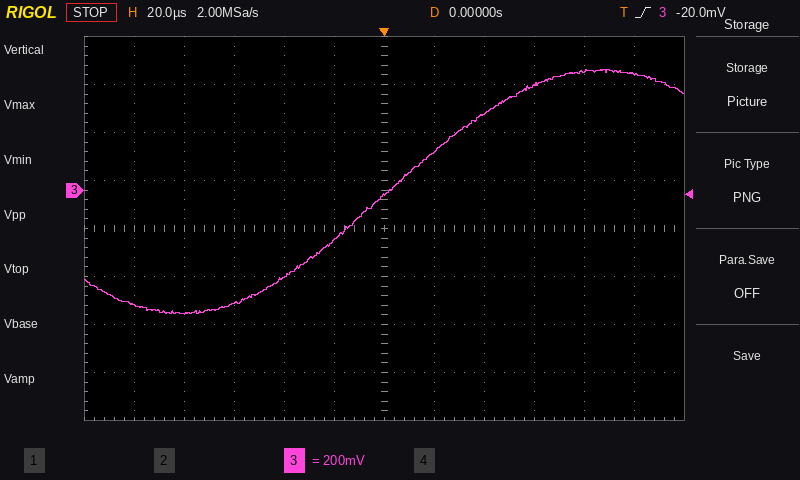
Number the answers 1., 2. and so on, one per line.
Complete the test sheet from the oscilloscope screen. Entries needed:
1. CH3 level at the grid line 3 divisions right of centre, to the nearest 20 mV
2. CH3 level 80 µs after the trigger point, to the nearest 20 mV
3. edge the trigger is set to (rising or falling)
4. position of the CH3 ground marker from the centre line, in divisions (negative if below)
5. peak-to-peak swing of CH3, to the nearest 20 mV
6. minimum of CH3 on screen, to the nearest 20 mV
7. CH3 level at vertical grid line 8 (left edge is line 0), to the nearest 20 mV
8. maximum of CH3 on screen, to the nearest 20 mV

1. 440 mV
2. 500 mV
3. rising
4. +0.8 div
5. 1.02 V
6. -520 mV
7. 320 mV
8. 500 mV
